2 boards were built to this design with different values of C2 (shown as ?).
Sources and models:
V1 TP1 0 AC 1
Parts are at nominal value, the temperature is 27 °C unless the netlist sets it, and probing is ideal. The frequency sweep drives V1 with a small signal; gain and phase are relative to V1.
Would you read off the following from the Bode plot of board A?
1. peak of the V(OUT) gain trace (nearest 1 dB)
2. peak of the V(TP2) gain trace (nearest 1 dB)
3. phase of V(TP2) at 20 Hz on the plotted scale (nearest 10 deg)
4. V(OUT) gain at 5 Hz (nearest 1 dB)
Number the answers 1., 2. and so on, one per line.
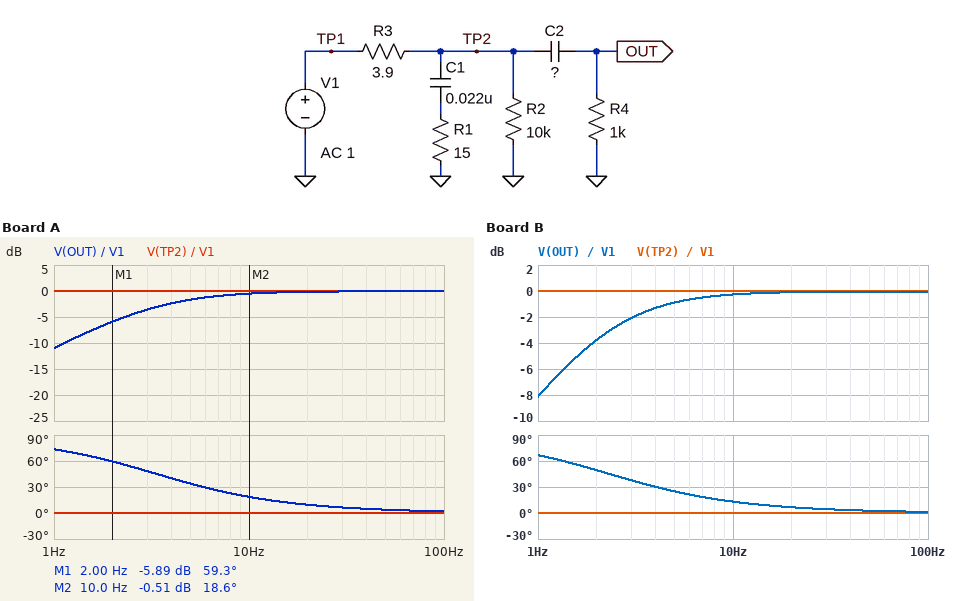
1. 0 dB
2. 0 dB
3. 0 deg
4. -2 dB
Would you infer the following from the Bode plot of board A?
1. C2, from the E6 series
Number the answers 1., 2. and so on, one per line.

1. 47 µF
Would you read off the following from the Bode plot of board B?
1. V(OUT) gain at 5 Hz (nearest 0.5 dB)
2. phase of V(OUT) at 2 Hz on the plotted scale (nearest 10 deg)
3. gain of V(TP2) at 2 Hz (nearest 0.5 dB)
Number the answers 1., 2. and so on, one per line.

1. -1.0 dB
2. 50 deg
3. 0 dB
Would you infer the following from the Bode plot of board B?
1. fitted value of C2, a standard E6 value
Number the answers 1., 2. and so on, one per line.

1. 68 µF
